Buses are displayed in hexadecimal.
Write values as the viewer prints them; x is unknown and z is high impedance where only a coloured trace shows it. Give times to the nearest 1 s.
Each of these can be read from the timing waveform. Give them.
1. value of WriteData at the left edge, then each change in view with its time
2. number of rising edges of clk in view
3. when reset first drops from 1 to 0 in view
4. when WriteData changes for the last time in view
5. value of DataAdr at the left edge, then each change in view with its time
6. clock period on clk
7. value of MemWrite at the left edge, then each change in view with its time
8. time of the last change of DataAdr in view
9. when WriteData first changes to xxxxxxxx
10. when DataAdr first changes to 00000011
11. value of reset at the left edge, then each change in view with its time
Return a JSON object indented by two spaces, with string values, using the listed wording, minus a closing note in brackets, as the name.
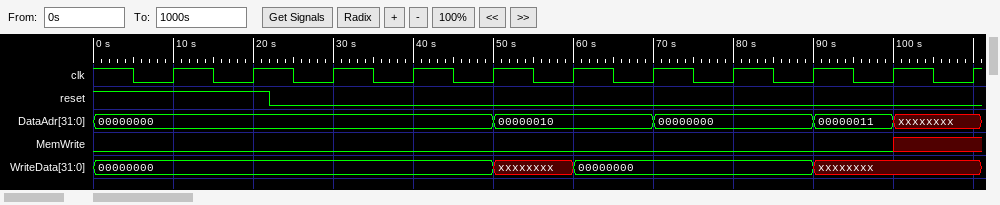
{
  "value of WriteData at the left edge, then each change in view with its time": "00000000, xxxxxxxx at 50 s, 00000000 at 60 s, xxxxxxxx at 90 s",
  "number of rising edges of clk in view": "11",
  "when reset first drops from 1 to 0 in view": "22 s",
  "when WriteData changes for the last time in view": "90 s",
  "value of DataAdr at the left edge, then each change in view with its time": "00000000, 00000010 at 50 s, 00000000 at 70 s, 00000011 at 90 s, xxxxxxxx at 100 s",
  "clock period on clk": "10 s",
  "value of MemWrite at the left edge, then each change in view with its time": "0, x at 100 s",
  "time of the last change of DataAdr in view": "100 s",
  "when WriteData first changes to xxxxxxxx": "50 s",
  "when DataAdr first changes to 00000011": "90 s",
  "value of reset at the left edge, then each change in view with its time": "1, 0 at 22 s"
}
